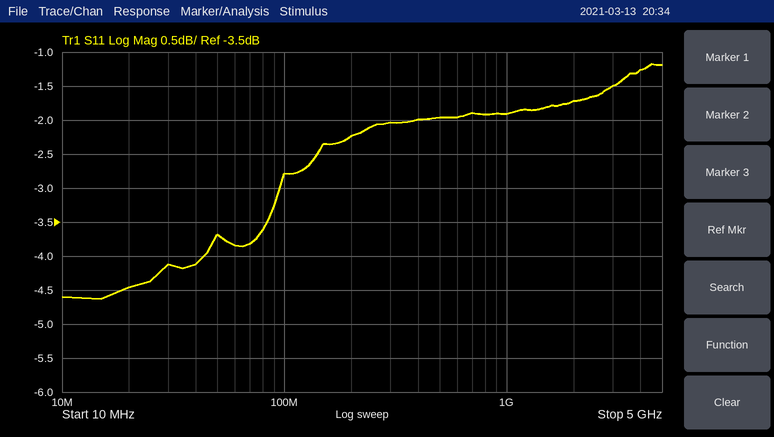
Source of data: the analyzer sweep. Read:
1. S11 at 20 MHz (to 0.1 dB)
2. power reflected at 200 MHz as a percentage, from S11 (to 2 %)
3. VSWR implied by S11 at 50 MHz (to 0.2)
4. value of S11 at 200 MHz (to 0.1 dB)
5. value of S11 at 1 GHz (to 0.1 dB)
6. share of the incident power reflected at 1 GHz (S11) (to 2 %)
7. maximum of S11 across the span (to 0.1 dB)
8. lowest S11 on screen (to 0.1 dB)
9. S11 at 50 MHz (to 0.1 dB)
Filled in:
-4.5 dB
60 %
4.8
-2.2 dB
-1.9 dB
64 %
-1.2 dB
-4.6 dB
-3.7 dB
